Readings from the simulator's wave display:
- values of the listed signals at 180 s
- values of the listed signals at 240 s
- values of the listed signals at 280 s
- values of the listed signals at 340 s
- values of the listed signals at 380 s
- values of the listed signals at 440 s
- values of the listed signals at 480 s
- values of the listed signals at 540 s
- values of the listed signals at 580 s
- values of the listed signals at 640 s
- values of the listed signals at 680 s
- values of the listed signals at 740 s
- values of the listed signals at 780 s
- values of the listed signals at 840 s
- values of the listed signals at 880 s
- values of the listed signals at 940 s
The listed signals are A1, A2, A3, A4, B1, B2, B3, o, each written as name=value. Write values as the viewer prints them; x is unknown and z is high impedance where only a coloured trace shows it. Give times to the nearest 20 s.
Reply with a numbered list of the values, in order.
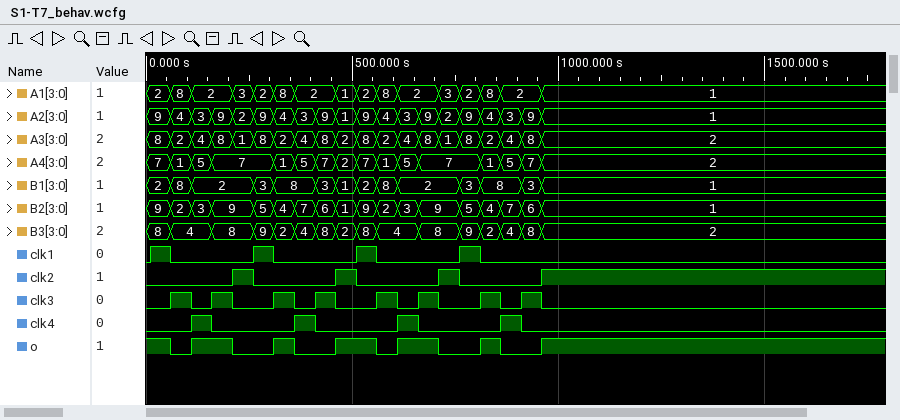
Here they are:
1. A1=2, A2=9, A3=8, A4=7, B1=2, B2=9, B3=8, o=1
2. A1=3, A2=2, A3=1, A4=7, B1=2, B2=9, B3=8, o=0
3. A1=2, A2=9, A3=8, A4=7, B1=3, B2=5, B3=9, o=0
4. A1=8, A2=4, A3=2, A4=1, B1=8, B2=4, B3=2, o=1
5. A1=2, A2=3, A3=4, A4=5, B1=8, B2=7, B3=4, o=0
6. A1=2, A2=9, A3=8, A4=7, B1=3, B2=6, B3=8, o=0
7. A1=1, A2=1, A3=2, A4=2, B1=1, B2=1, B3=2, o=1
8. A1=2, A2=9, A3=8, A4=7, B1=2, B2=9, B3=8, o=1
9. A1=8, A2=4, A3=2, A4=1, B1=8, B2=2, B3=4, o=0
10. A1=2, A2=3, A3=4, A4=5, B1=2, B2=3, B3=4, o=1
11. A1=2, A2=9, A3=8, A4=7, B1=2, B2=9, B3=8, o=1
12. A1=3, A2=2, A3=1, A4=7, B1=2, B2=9, B3=8, o=0
13. A1=2, A2=9, A3=8, A4=7, B1=3, B2=5, B3=9, o=0
14. A1=8, A2=4, A3=2, A4=1, B1=8, B2=4, B3=2, o=1
15. A1=2, A2=3, A3=4, A4=5, B1=8, B2=7, B3=4, o=0
16. A1=2, A2=9, A3=8, A4=7, B1=3, B2=6, B3=8, o=0
